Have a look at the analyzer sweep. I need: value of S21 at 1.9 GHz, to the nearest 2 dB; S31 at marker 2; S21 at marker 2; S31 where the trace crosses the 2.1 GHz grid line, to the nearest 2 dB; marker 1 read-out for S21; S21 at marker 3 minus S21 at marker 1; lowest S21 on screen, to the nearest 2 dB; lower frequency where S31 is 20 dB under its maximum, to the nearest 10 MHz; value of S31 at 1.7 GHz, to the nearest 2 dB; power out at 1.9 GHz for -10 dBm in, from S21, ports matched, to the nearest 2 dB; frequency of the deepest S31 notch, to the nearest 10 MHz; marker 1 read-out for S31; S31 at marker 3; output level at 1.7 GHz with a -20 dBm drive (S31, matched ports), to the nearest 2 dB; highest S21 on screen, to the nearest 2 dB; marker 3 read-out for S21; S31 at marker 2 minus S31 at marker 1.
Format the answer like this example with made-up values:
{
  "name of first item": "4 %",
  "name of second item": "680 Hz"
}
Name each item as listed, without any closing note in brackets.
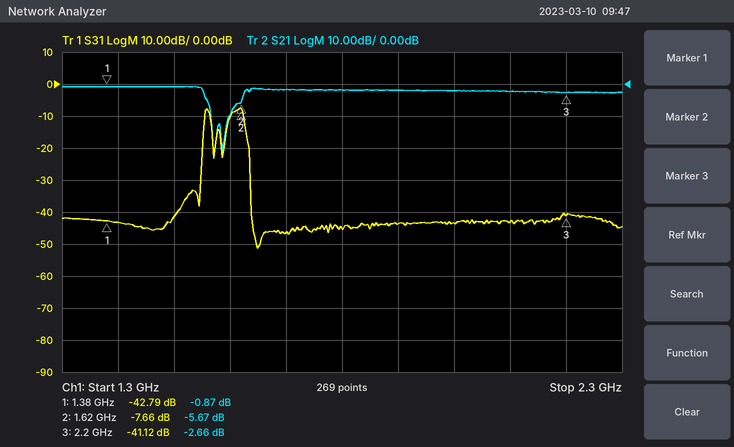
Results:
{
  "value of S21 at 1.9 GHz, to the nearest 2 dB": "-2 dB",
  "S31 at marker 2": "-7.66 dB",
  "S21 at marker 2": "-5.67 dB",
  "S31 where the trace crosses the 2.1 GHz grid line, to the nearest 2 dB": "-44 dB",
  "marker 1 read-out for S21": "-0.87 dB",
  "S21 at marker 3 minus S21 at marker 1": "-1.79 dB",
  "lowest S21 on screen, to the nearest 2 dB": "-24 dB",
  "lower frequency where S31 is 20 dB under its maximum, to the nearest 10 MHz": "1.55 GHz",
  "value of S31 at 1.7 GHz, to the nearest 2 dB": "-46 dB",
  "power out at 1.9 GHz for -10 dBm in, from S21, ports matched, to the nearest 2 dB": "-12 dBm",
  "frequency of the deepest S31 notch, to the nearest 10 MHz": "1.65 GHz",
  "marker 1 read-out for S31": "-42.79 dB",
  "S31 at marker 3": "-41.12 dB",
  "output level at 1.7 GHz with a -20 dBm drive (S31, matched ports), to the nearest 2 dB": "-66 dBm",
  "highest S21 on screen, to the nearest 2 dB": "0 dB",
  "marker 3 read-out for S21": "-2.66 dB",
  "S31 at marker 2 minus S31 at marker 1": "35.13 dB"
}
